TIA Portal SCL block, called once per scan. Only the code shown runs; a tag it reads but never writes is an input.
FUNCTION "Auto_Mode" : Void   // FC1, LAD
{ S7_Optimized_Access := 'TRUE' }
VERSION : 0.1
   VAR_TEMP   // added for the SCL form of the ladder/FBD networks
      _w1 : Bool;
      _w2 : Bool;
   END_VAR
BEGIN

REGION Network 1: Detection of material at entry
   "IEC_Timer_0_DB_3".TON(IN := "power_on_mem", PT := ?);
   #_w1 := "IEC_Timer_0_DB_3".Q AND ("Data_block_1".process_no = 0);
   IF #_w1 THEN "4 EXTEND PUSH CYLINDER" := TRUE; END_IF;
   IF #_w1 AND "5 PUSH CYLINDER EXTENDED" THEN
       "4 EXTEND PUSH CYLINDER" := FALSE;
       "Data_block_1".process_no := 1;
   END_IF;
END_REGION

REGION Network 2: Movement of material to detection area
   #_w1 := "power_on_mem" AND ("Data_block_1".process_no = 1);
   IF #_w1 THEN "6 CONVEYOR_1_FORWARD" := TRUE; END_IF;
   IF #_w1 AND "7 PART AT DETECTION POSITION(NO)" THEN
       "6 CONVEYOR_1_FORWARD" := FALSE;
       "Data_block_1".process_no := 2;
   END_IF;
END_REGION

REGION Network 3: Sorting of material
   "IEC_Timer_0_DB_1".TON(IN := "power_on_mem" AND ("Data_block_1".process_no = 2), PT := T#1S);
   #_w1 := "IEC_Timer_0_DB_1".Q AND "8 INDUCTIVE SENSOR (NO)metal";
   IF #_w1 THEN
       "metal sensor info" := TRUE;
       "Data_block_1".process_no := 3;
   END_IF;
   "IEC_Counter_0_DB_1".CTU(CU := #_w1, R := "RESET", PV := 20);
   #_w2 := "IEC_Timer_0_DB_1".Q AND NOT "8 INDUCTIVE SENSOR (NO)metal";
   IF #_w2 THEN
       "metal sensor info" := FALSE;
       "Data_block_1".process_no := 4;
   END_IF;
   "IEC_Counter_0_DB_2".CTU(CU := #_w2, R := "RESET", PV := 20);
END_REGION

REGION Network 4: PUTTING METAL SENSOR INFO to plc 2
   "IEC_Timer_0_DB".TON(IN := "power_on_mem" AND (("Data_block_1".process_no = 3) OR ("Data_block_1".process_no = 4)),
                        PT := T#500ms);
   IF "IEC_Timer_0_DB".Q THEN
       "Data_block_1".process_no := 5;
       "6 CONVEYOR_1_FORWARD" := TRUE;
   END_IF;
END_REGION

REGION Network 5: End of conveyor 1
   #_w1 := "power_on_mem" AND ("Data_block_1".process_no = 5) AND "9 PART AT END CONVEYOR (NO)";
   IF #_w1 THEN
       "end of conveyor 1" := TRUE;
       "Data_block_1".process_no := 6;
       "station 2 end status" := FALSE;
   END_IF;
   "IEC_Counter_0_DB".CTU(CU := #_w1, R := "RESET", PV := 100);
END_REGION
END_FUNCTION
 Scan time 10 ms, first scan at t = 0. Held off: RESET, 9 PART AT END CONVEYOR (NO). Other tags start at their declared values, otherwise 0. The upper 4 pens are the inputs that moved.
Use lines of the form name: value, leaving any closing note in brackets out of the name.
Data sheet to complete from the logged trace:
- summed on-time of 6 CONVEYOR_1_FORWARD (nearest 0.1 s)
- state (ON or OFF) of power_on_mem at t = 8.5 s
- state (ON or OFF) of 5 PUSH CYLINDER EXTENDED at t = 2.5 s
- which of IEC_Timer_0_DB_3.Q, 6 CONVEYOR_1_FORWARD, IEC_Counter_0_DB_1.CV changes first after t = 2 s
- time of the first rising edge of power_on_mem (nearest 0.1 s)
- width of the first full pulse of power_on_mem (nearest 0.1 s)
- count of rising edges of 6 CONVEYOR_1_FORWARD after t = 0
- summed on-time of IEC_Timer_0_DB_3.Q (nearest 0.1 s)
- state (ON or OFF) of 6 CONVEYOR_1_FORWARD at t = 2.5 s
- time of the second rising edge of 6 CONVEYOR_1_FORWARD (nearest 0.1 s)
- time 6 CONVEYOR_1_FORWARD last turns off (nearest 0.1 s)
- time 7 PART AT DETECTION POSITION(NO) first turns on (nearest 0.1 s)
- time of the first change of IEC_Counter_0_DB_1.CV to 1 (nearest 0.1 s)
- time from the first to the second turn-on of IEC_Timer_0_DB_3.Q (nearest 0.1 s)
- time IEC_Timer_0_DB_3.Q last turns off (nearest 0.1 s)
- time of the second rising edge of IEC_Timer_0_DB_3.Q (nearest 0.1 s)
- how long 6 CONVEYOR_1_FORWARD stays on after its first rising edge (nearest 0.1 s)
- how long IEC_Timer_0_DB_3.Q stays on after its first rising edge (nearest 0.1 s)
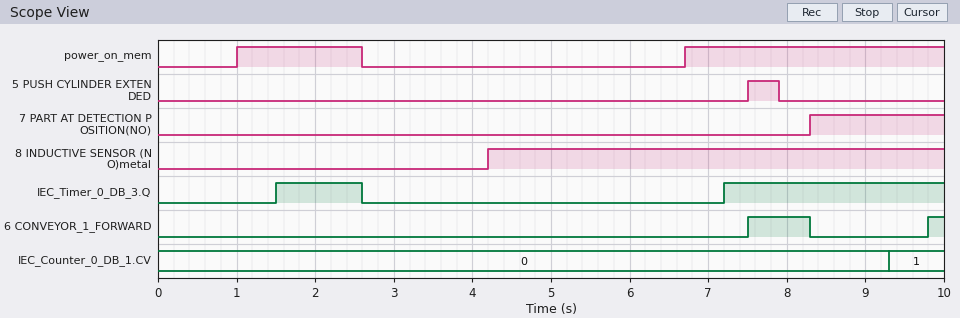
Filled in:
summed on-time of 6 CONVEYOR_1_FORWARD: 1.0 s
state (ON or OFF) of power_on_mem at t = 8.5 s: ON
state (ON or OFF) of 5 PUSH CYLINDER EXTENDED at t = 2.5 s: OFF
which of IEC_Timer_0_DB_3.Q, 6 CONVEYOR_1_FORWARD, IEC_Counter_0_DB_1.CV changes first after t = 2 s: IEC_Timer_0_DB_3.Q
time of the first rising edge of power_on_mem: 1.0 s
width of the first full pulse of power_on_mem: 1.6 s
count of rising edges of 6 CONVEYOR_1_FORWARD after t = 0: 2
summed on-time of IEC_Timer_0_DB_3.Q: 3.9 s
state (ON or OFF) of 6 CONVEYOR_1_FORWARD at t = 2.5 s: OFF
time of the second rising edge of 6 CONVEYOR_1_FORWARD: 9.8 s
time 6 CONVEYOR_1_FORWARD last turns off: 8.3 s
time 7 PART AT DETECTION POSITION(NO) first turns on: 8.3 s
time of the first change of IEC_Counter_0_DB_1.CV to 1: 9.3 s
time from the first to the second turn-on of IEC_Timer_0_DB_3.Q: 5.7 s
time IEC_Timer_0_DB_3.Q last turns off: 2.6 s
time of the second rising edge of IEC_Timer_0_DB_3.Q: 7.2 s
how long 6 CONVEYOR_1_FORWARD stays on after its first rising edge: 0.8 s
how long IEC_Timer_0_DB_3.Q stays on after its first rising edge: 1.1 s
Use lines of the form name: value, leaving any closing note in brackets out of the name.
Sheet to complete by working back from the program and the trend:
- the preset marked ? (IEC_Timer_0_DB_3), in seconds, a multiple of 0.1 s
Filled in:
the preset marked ? (IEC_Timer_0_DB_3), in seconds, a multiple of 0.1 s: 0.5 s
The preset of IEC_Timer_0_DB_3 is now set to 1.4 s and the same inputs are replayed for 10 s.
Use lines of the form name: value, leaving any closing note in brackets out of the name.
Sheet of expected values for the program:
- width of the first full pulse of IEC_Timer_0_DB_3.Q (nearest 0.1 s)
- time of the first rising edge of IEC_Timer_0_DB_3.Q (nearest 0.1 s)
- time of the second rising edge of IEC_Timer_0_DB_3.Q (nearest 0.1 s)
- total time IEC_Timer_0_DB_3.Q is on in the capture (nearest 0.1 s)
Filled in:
width of the first full pulse of IEC_Timer_0_DB_3.Q: 0.2 s
time of the first rising edge of IEC_Timer_0_DB_3.Q: 2.4 s
time of the second rising edge of IEC_Timer_0_DB_3.Q: 8.1 s
total time IEC_Timer_0_DB_3.Q is on in the capture: 2.1 s
